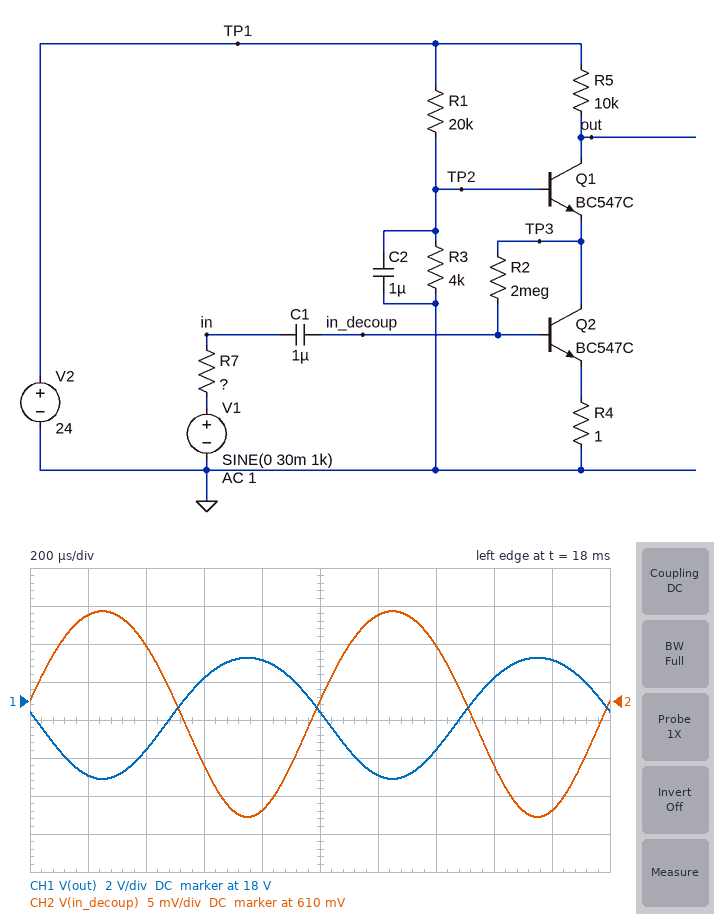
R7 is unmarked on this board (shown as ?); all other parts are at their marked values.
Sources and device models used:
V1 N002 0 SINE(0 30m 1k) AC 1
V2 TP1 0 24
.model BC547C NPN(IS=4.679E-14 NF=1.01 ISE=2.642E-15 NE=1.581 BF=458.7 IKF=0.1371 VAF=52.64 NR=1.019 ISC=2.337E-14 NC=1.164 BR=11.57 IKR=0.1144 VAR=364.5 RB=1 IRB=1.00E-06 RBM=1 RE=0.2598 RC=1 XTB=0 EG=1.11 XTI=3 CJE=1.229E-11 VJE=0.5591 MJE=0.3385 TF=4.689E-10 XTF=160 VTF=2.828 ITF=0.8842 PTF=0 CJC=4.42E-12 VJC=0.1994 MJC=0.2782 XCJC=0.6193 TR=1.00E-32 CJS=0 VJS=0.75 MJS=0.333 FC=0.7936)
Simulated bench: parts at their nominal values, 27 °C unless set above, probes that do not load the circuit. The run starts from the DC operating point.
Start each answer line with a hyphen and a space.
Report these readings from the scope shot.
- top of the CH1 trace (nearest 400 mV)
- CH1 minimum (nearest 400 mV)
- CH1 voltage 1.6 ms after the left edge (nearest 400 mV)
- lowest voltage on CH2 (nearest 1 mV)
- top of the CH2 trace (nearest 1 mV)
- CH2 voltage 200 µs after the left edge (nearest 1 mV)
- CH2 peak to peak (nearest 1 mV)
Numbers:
- 20.4 V
- 14.0 V
- 19.2 V
- 595 mV
- 622 mV
- 621 mV
- 27 mV
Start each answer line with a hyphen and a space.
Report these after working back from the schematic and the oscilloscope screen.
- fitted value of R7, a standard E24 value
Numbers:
- 24 kΩ
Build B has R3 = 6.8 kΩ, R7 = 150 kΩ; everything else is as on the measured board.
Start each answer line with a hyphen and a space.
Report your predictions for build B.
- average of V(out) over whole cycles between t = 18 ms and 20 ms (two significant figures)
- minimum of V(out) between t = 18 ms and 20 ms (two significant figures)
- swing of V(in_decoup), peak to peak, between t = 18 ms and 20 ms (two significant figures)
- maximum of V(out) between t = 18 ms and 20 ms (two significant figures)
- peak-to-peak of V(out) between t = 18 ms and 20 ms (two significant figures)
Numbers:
- 12 V
- 11 V
- 4.2 mV
- 13 V
- 1.8 V
